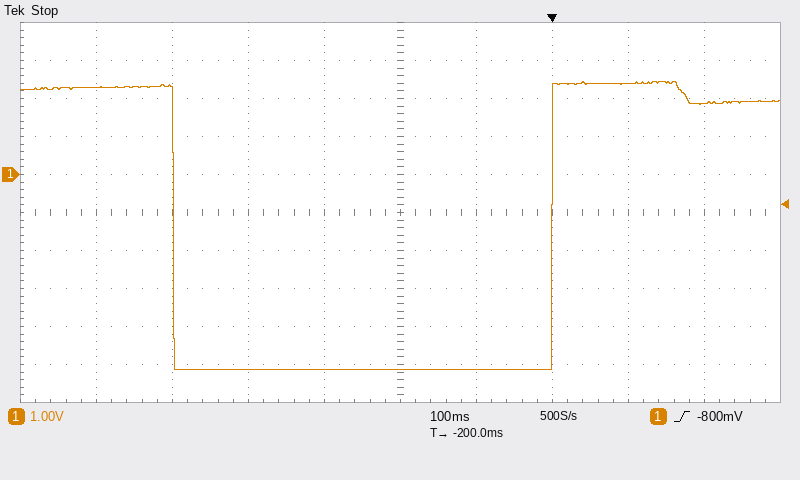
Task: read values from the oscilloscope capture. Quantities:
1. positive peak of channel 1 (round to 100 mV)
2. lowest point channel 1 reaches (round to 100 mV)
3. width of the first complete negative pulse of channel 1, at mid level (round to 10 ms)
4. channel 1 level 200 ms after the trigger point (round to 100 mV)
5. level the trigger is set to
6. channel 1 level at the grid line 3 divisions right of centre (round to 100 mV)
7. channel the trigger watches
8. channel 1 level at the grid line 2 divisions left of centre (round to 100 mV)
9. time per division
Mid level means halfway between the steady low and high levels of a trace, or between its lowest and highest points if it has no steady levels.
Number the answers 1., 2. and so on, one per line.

1. 2.4 V
2. -5.1 V
3. 500 ms
4. 1.9 V
5. -800 mV
6. 2.4 V
7. channel 1
8. -5.1 V
9. 100 ms
